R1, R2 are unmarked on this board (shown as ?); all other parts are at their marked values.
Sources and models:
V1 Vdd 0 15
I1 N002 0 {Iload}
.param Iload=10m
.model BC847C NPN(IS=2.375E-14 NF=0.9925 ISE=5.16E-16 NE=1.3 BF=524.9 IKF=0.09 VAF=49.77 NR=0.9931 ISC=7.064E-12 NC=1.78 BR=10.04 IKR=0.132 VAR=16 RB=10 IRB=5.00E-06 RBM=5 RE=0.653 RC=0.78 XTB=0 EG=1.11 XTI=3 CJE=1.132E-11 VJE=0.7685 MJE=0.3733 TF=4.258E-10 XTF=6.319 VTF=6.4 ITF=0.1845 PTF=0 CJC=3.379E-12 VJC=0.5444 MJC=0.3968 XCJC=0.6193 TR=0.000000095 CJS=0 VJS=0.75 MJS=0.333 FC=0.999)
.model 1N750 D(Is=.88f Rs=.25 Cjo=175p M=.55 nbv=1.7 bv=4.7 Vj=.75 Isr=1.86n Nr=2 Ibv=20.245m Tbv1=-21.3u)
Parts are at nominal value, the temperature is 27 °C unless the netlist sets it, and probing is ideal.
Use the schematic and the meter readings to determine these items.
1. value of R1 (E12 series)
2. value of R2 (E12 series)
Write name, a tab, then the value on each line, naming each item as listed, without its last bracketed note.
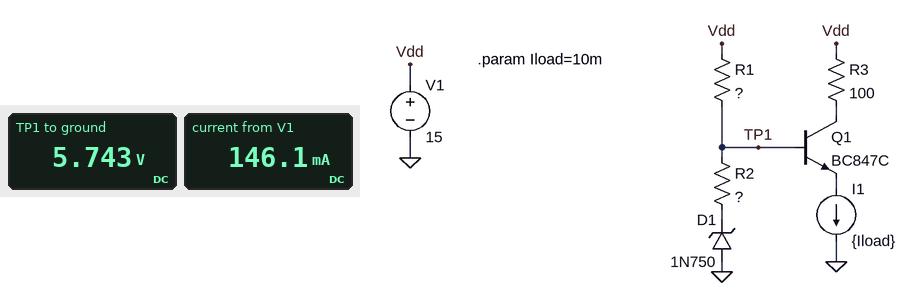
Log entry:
value of R1	68 Ω
value of R2	6.8 Ω
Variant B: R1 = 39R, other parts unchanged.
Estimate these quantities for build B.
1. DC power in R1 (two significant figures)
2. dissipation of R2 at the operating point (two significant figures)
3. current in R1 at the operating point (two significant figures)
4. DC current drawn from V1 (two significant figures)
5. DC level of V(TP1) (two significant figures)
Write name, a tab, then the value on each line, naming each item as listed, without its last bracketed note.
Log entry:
DC power in R1	1.9 W
dissipation of R2 at the operating point	330 mW
current in R1 at the operating point	220 mA
DC current drawn from V1	230 mA
DC level of V(TP1)	6.4 V
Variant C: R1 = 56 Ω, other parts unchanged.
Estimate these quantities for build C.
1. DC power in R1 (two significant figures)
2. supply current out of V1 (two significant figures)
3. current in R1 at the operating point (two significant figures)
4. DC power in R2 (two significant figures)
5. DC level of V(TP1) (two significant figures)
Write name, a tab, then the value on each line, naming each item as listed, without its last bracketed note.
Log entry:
DC power in R1	1.5 W
supply current out of V1	170 mA
current in R1 at the operating point	160 mA
DC power in R2	180 mW
DC level of V(TP1)	5.9 V
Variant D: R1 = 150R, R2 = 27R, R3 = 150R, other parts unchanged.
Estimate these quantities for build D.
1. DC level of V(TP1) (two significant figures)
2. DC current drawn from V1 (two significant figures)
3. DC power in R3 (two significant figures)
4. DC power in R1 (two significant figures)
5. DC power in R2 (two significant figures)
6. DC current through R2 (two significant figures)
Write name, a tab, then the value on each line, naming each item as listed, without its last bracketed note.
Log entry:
DC level of V(TP1)	6.3 V
DC current drawn from V1	68 mA
DC power in R3	15 mW
DC power in R1	500 mW
DC power in R2	90 mW
DC current through R2	58 mA
